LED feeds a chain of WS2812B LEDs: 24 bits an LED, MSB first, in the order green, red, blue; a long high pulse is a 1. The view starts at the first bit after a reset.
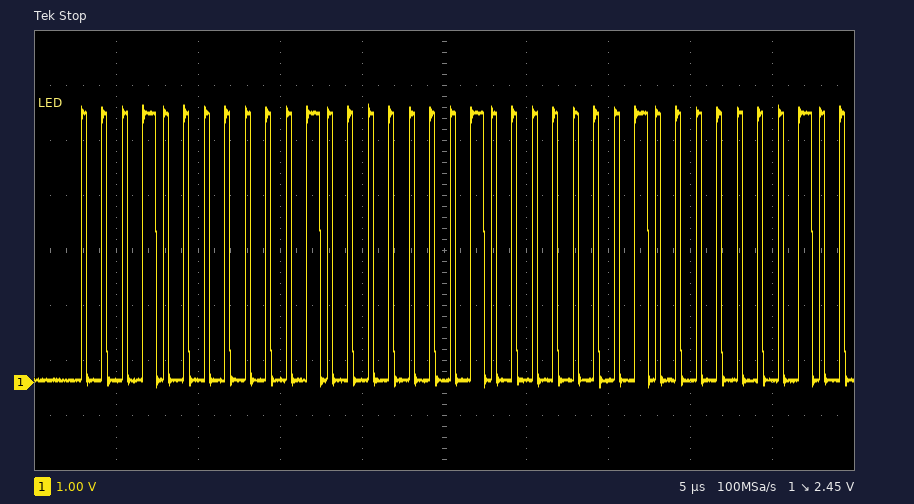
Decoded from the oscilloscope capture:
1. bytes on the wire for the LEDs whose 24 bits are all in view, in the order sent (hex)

10 10 10
